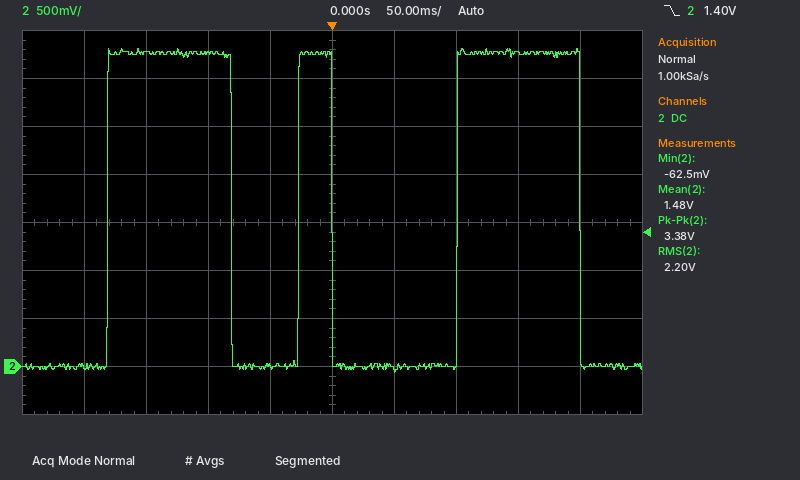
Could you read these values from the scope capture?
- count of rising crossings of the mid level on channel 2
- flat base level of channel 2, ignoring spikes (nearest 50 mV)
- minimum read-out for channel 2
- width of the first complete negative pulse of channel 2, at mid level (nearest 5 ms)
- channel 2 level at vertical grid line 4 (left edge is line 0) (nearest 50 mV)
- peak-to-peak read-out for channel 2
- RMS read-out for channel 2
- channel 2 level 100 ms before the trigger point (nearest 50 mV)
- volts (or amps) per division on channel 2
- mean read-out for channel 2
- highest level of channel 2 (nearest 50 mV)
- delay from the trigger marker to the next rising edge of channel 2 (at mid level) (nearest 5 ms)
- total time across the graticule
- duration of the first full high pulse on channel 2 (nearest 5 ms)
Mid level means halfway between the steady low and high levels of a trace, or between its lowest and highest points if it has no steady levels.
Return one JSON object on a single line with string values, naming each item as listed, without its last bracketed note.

{"count of rising crossings of the mid level on channel 2": "3", "flat base level of channel 2, ignoring spikes": "0 mV", "minimum read-out for channel 2": "-62.5 mV", "width of the first complete negative pulse of channel 2, at mid level": "55 ms", "channel 2 level at vertical grid line 4 (left edge is line 0)": "0 mV", "peak-to-peak read-out for channel 2": "3.38 V", "RMS read-out for channel 2": "2.20 V", "channel 2 level 100 ms before the trigger point": "3.25 V", "volts (or amps) per division on channel 2": "500 mV", "mean read-out for channel 2": "1.48 V", "highest level of channel 2": "3.30 V", "delay from the trigger marker to the next rising edge of channel 2 (at mid level)": "100 ms", "total time across the graticule": "500 ms", "duration of the first full high pulse on channel 2": "100 ms"}
